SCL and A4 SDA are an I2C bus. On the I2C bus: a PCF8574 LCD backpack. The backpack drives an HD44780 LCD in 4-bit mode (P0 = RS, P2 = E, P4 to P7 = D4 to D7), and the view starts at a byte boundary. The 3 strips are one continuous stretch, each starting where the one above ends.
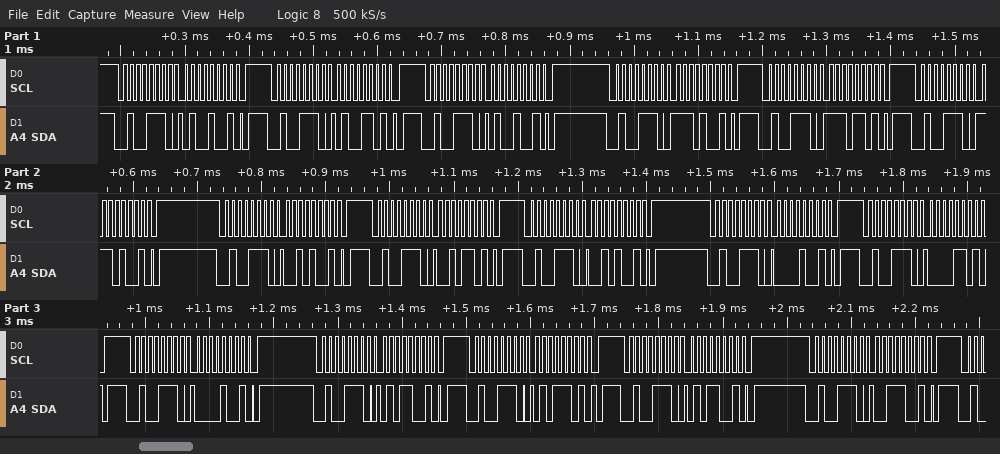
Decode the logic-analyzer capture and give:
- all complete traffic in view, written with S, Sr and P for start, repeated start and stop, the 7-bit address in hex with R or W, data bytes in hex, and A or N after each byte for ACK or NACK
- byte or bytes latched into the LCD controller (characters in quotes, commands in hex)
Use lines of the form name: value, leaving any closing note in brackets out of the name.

all complete traffic in view, written with S, Sr and P for start, repeated start and stop, the 7-bit address in hex with R or W, data bytes in hex, and A or N after each byte for ACK or NACK: S 27W A 49 A P S 27W A 4D A P S 27W A 49 A P S 27W A E9 A P S 27W A ED A P S 27W A E9 A P S 27W A 29 A P S 27W A 2D A P S 27W A 29 A P S 27W A 09 A P S 27W A 0D A P S 27W A 09 A P S 27W A 59 A P S 27W A 5D A P S 27W A 59 A P S 27W A 39 A P
byte or bytes latched into the LCD controller: 'N' ' '
